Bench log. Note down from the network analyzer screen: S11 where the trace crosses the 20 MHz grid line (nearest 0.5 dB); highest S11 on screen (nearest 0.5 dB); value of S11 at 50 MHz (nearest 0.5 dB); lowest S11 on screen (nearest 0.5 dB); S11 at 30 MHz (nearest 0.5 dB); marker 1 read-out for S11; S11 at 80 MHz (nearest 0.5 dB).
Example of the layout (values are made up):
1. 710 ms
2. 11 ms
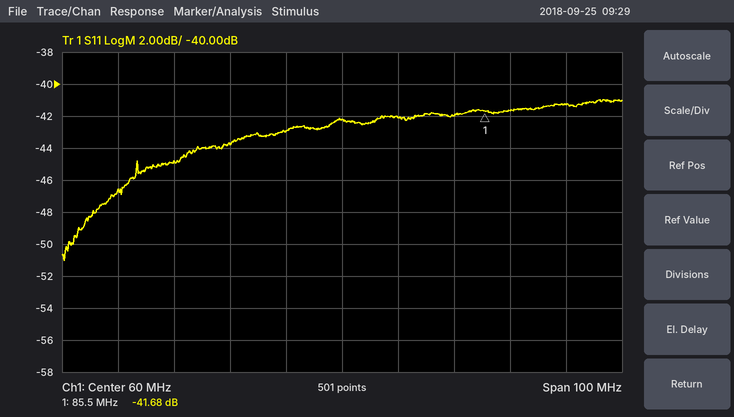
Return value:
1. -46.5 dB
2. -41.0 dB
3. -43.0 dB
4. -51.0 dB
5. -45.0 dB
6. -41.68 dB
7. -42.0 dB
